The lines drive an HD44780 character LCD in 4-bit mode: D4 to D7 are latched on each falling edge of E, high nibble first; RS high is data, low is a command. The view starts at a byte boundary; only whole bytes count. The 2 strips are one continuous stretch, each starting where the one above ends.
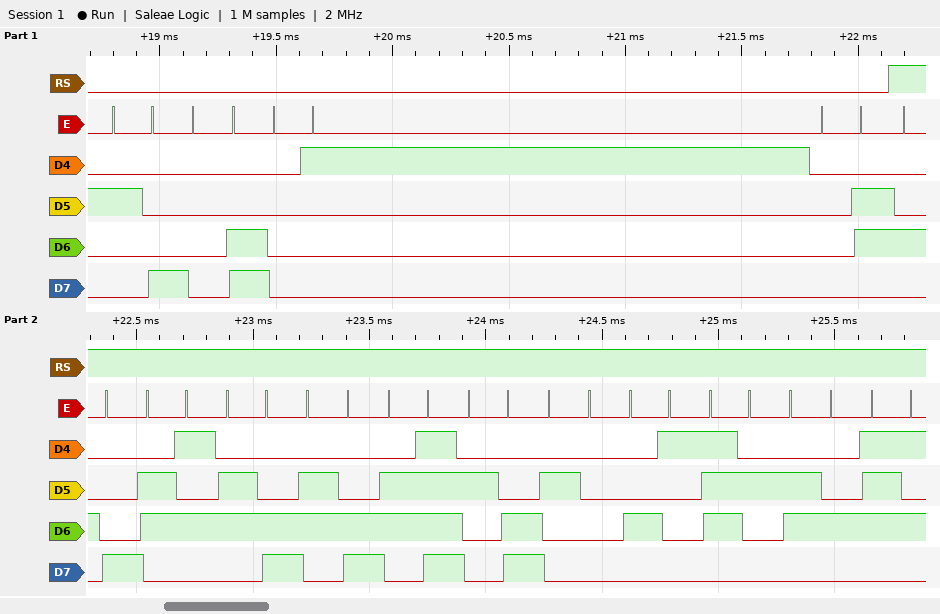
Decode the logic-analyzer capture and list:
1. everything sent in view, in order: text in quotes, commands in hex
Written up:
0x28 0x0C 0x01 0x06 "Hello, Ardu"
